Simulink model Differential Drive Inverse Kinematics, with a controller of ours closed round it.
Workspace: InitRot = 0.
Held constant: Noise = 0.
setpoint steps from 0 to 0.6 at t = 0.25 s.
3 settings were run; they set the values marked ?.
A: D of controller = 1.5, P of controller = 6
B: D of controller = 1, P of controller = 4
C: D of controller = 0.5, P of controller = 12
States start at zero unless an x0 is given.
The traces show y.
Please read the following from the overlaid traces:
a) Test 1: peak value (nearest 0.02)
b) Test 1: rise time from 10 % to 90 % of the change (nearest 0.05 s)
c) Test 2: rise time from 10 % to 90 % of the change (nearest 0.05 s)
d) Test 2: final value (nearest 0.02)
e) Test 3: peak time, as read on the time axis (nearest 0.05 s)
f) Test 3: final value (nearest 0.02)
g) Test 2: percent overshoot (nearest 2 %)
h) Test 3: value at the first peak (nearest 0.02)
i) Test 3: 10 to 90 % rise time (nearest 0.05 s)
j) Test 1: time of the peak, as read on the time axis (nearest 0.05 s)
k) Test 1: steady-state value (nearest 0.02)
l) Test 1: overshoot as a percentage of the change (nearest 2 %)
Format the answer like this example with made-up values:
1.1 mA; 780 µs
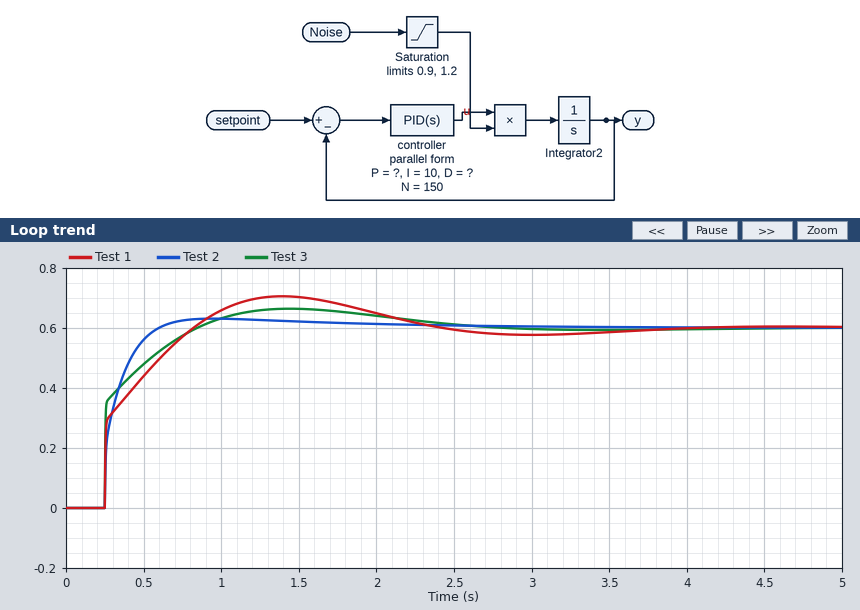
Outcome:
0.70; 0.45 s; 0.20 s; 0.60; 1.45 s; 0.60; 6 %; 0.66; 0.40 s; 1.40 s; 0.60; 18 %
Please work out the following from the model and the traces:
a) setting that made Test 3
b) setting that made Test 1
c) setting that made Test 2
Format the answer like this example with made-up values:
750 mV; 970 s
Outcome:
A; B; C
